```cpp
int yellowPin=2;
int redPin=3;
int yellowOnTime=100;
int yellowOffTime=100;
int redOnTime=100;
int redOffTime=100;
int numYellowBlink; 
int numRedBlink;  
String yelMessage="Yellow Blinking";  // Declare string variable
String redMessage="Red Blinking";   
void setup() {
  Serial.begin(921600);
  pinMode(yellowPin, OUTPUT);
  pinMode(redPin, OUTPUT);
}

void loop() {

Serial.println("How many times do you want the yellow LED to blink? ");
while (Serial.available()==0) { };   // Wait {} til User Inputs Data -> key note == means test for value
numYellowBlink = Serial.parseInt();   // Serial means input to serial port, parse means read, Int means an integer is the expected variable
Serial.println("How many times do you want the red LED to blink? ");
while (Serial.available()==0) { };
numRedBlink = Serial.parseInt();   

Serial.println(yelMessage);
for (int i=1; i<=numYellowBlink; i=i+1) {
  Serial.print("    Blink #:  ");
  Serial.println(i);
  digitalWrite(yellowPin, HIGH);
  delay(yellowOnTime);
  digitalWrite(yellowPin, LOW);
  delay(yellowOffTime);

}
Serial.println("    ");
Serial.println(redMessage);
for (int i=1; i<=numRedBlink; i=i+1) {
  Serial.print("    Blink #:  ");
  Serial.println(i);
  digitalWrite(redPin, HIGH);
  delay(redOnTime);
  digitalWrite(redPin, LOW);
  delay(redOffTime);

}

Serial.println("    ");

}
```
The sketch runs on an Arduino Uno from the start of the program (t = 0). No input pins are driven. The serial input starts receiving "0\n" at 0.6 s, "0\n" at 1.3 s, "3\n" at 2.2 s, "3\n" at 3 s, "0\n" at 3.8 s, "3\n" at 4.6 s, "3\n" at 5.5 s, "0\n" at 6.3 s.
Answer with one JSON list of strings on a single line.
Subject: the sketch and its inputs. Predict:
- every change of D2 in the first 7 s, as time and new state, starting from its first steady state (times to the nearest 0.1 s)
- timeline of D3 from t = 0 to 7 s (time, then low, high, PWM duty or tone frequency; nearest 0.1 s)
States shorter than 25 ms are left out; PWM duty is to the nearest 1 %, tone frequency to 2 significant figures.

["0 s low; 3 s high; 3.1 s low; 3.2 s high; 3.3 s low; 3.4 s high; 3.5 s low; 6.3 s high; 6.4 s low; 6.5 s high; 6.6 s low; 6.7 s high; 6.8 s low", "0 s low; 3.6 s high; 3.7 s low; 3.8 s high; 3.9 s low; 4 s high; 4.1 s low; 4.6 s high; 4.7 s low; 4.8 s high; 4.9 s low; 5 s high; 5.1 s low"]
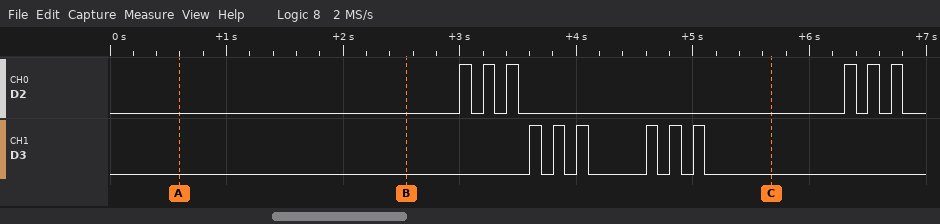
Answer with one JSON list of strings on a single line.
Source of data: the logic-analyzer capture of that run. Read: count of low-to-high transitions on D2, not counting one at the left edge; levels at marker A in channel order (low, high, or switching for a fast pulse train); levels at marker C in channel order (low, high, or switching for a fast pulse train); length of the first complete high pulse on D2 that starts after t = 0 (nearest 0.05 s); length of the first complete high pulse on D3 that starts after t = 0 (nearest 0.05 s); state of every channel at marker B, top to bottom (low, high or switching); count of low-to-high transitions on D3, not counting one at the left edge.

["6", "D2 low, D3 low", "D2 low, D3 low", "0.10 s", "0.10 s", "D2 low, D3 low", "6"]
